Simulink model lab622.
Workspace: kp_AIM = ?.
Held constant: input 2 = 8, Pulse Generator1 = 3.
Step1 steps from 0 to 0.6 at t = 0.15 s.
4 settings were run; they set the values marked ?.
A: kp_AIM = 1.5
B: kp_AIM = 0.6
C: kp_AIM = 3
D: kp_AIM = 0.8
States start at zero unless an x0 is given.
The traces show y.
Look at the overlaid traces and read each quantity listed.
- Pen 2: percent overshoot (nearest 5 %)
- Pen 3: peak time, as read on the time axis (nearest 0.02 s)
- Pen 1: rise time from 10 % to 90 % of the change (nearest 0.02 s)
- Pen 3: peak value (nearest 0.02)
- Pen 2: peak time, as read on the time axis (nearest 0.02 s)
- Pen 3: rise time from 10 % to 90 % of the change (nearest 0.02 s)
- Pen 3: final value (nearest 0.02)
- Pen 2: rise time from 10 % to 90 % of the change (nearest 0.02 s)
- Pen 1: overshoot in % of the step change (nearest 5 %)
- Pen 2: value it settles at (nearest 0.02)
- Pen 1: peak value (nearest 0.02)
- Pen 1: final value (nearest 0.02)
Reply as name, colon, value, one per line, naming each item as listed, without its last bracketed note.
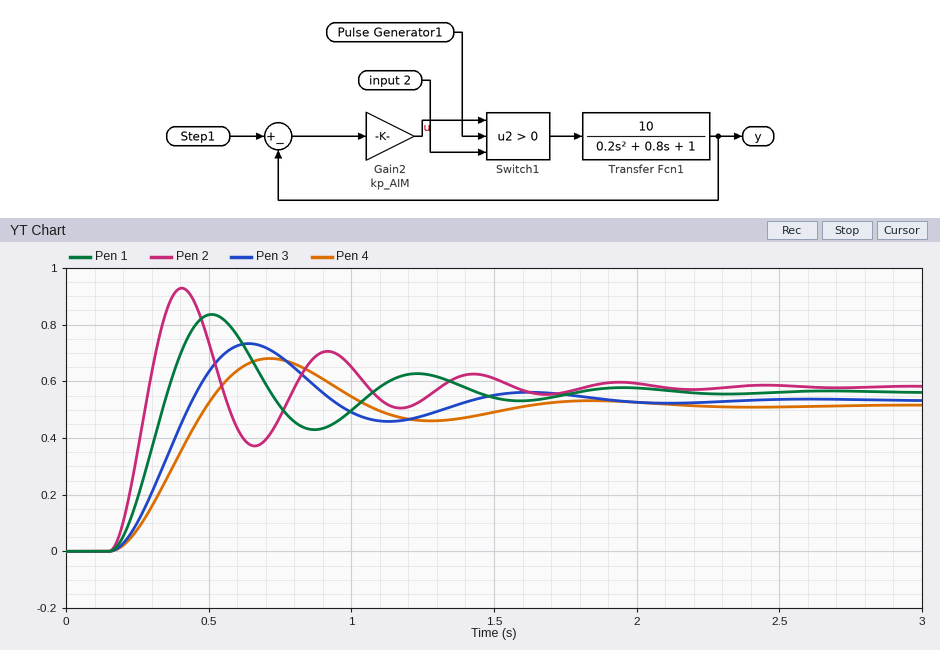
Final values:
Pen 2: percent overshoot: 60 %
Pen 3: peak time, as read on the time axis: 0.64 s
Pen 1: rise time from 10 % to 90 % of the change: 0.14 s
Pen 3: peak value: 0.74
Pen 2: peak time, as read on the time axis: 0.40 s
Pen 3: rise time from 10 % to 90 % of the change: 0.20 s
Pen 3: final value: 0.54
Pen 2: rise time from 10 % to 90 % of the change: 0.10 s
Pen 1: overshoot in % of the step change: 50 %
Pen 2: value it settles at: 0.58
Pen 1: peak value: 0.84
Pen 1: final value: 0.56
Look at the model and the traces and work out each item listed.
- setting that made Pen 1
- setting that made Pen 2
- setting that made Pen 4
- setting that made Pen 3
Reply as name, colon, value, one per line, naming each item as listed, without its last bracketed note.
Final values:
setting that made Pen 1: A
setting that made Pen 2: C
setting that made Pen 4: B
setting that made Pen 3: D
